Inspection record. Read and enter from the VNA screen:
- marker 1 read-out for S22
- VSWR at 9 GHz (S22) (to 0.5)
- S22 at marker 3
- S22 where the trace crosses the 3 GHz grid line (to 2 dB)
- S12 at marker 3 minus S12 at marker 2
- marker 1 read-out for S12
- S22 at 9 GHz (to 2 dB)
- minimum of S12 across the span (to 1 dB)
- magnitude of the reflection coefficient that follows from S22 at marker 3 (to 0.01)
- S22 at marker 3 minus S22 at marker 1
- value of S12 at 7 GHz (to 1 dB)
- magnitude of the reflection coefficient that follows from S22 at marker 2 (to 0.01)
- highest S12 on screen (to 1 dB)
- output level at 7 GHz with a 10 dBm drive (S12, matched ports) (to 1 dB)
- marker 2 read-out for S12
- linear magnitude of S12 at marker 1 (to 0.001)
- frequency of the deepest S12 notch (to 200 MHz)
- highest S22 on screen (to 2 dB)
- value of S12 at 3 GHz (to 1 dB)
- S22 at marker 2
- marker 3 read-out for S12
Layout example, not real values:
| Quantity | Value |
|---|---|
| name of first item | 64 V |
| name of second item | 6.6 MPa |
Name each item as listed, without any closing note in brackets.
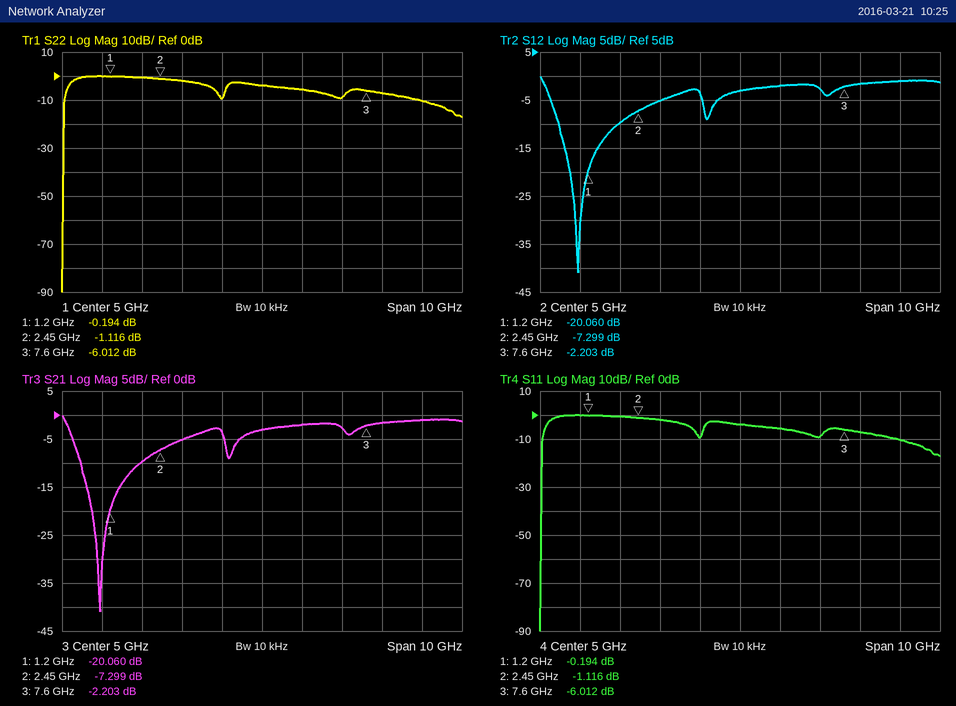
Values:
| Quantity | Value |
|---|---|
| marker 1 read-out for S22 | -0.194 dB |
| VSWR at 9 GHz (S22) | 2.0 |
| S22 at marker 3 | -6.012 dB |
| S22 where the trace crosses the 3 GHz grid line | -2 dB |
| S12 at marker 3 minus S12 at marker 2 | 5.096 dB |
| marker 1 read-out for S12 | -20.060 dB |
| S22 at 9 GHz | -10 dB |
| minimum of S12 across the span | -41 dB |
| magnitude of the reflection coefficient that follows from S22 at marker 3 | 0.50 |
| S22 at marker 3 minus S22 at marker 1 | -5.818 dB |
| value of S12 at 7 GHz | -3 dB |
| magnitude of the reflection coefficient that follows from S22 at marker 2 | 0.88 |
| highest S12 on screen | 0 dB |
| output level at 7 GHz with a 10 dBm drive (S12, matched ports) | 7 dBm |
| marker 2 read-out for S12 | -7.299 dB |
| linear magnitude of S12 at marker 1 | 0.099 |
| frequency of the deepest S12 notch | 1.0 GHz |
| highest S22 on screen | 0 dB |
| value of S12 at 3 GHz | -5 dB |
| S22 at marker 2 | -1.116 dB |
| marker 3 read-out for S12 | -2.203 dB |
